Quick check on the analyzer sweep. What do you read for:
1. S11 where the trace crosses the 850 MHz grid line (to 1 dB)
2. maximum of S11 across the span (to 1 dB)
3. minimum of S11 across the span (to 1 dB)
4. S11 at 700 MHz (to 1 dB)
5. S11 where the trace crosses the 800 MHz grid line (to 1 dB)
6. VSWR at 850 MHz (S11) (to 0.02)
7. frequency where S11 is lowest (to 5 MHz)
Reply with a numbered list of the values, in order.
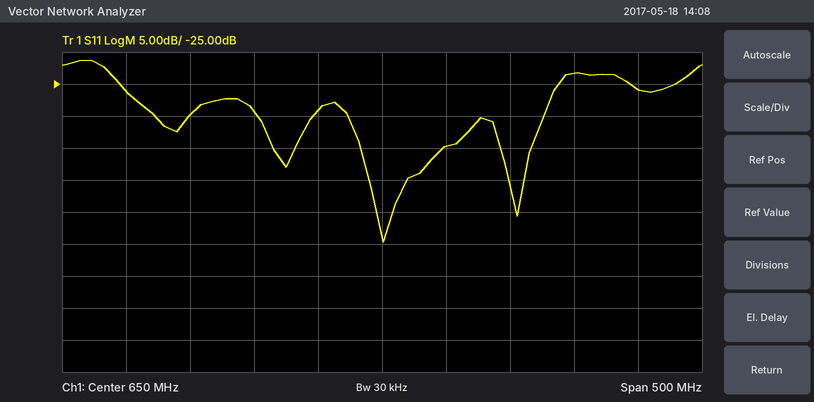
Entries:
1. -26 dB
2. -21 dB
3. -50 dB
4. -35 dB
5. -23 dB
6. 1.10
7. 650 MHz
